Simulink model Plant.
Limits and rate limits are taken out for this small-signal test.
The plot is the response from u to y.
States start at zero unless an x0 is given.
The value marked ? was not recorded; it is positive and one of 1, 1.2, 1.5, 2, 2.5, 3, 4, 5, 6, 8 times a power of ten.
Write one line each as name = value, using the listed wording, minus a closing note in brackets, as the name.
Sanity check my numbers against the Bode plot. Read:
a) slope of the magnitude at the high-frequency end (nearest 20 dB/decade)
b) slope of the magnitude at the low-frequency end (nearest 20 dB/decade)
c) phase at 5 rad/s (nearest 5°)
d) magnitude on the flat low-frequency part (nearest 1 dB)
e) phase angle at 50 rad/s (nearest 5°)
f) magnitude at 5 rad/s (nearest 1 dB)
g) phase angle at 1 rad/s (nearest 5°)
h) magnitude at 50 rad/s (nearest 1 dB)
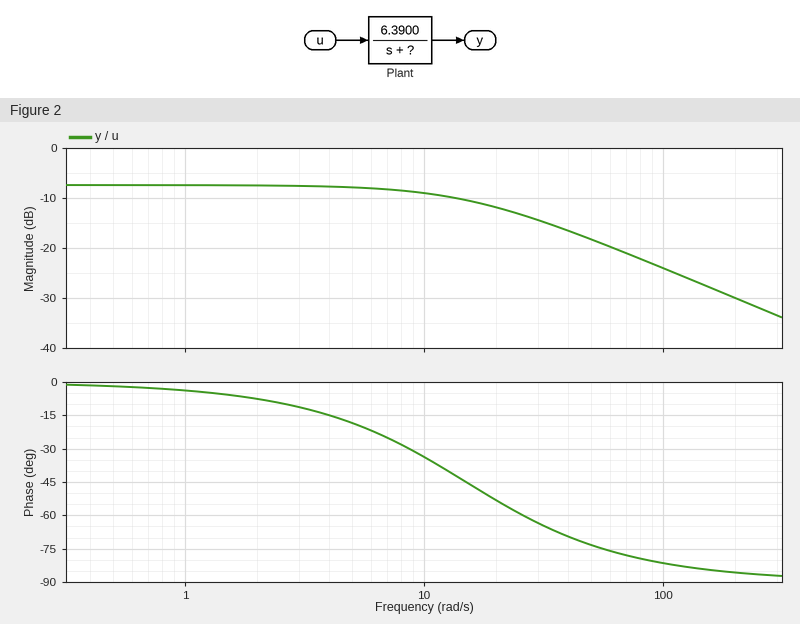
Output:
slope of the magnitude at the high-frequency end = -20 dB/decade
slope of the magnitude at the low-frequency end = 0 dB/decade
phase at 5 rad/s = -20°
magnitude on the flat low-frequency part = -7 dB
phase angle at 50 rad/s = -75°
magnitude at 5 rad/s = -8 dB
phase angle at 1 rad/s = -5°
magnitude at 50 rad/s = -18 dB
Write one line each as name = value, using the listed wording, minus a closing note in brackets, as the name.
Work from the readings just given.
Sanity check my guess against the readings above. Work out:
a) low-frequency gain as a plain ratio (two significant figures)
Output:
low-frequency gain as a plain ratio = 0.45
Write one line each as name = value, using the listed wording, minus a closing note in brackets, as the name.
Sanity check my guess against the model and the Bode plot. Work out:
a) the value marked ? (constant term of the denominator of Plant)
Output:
the value marked ? = 15
